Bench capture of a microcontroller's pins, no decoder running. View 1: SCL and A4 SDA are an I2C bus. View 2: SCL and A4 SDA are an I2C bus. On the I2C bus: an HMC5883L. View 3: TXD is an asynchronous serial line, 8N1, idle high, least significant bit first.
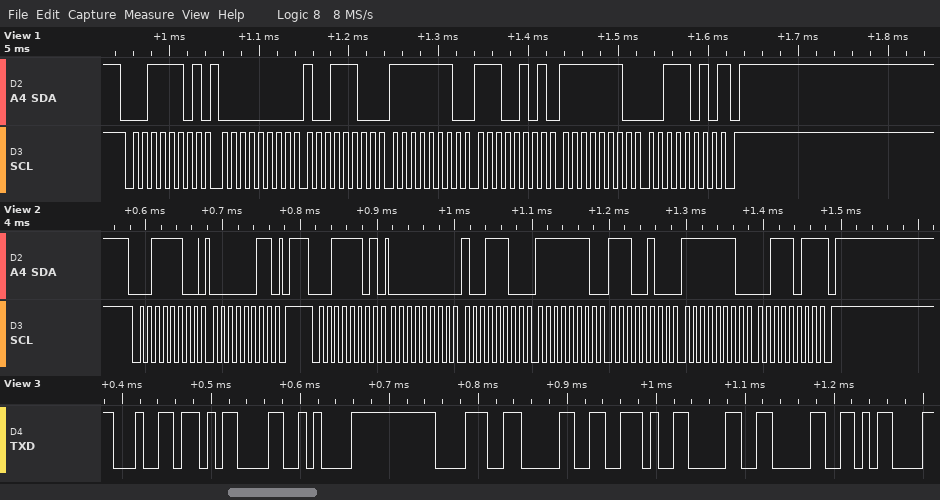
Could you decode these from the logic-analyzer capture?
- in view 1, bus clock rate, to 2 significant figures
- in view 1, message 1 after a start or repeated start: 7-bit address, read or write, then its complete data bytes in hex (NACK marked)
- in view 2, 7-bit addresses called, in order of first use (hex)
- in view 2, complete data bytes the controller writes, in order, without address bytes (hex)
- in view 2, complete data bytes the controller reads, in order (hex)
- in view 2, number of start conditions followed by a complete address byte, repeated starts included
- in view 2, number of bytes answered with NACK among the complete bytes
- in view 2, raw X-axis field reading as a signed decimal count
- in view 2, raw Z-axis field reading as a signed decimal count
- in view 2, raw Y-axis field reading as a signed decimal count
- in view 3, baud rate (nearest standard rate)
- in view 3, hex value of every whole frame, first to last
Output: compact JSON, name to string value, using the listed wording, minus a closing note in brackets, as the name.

{"in view 1, bus clock rate, to 2 significant figures": "100 kHz", "in view 1, message 1 after a start or repeated start: 7-bit address, read or write, then its complete data bytes in hex": "0x1E read: 00 9C FE E5 FE 3A NACK", "in view 2, 7-bit addresses called, in order of first use": "0x1E", "in view 2, complete data bytes the controller writes, in order, without address bytes": "03", "in view 2, complete data bytes the controller reads, in order": "00 9C FE E4 FE 3B", "in view 2, number of start conditions followed by a complete address byte, repeated starts included": "2", "in view 2, number of bytes answered with NACK among the complete bytes": "1", "in view 2, raw X-axis field reading as a signed decimal count": "156", "in view 2, raw Z-axis field reading as a signed decimal count": "-284", "in view 2, raw Y-axis field reading as a signed decimal count": "-453", "in view 3, baud rate": "115200 baud", "in view 3, hex value of every whole frame, first to last": "64 0D 0A 38 30 2E 30 30 0D"}
